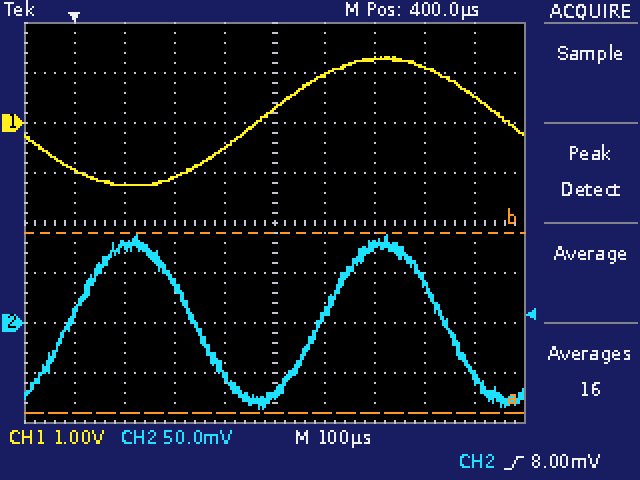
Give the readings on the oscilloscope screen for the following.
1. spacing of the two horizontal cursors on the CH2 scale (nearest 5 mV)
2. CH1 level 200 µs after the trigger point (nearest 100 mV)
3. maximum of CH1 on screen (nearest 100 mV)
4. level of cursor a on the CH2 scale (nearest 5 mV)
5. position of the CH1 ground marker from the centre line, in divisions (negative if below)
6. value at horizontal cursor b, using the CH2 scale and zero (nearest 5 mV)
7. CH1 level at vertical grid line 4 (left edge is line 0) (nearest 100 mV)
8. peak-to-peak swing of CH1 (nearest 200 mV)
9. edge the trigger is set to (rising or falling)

180 mV
-1.1 V
1.3 V
-90 mV
+2.0 div
90 mV
-500 mV
2.6 V
rising
